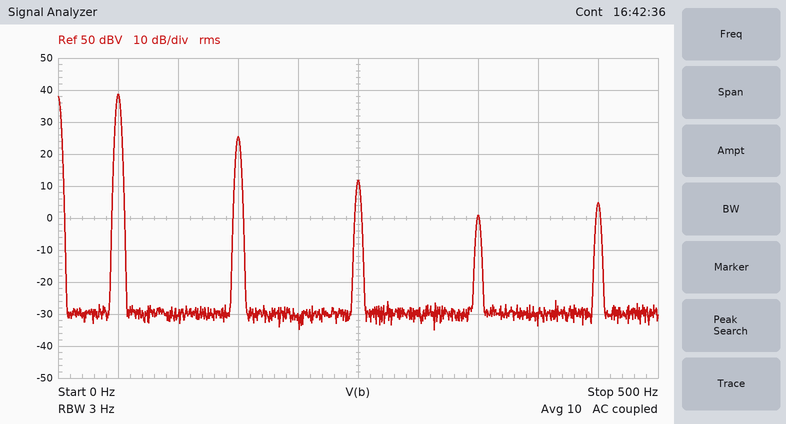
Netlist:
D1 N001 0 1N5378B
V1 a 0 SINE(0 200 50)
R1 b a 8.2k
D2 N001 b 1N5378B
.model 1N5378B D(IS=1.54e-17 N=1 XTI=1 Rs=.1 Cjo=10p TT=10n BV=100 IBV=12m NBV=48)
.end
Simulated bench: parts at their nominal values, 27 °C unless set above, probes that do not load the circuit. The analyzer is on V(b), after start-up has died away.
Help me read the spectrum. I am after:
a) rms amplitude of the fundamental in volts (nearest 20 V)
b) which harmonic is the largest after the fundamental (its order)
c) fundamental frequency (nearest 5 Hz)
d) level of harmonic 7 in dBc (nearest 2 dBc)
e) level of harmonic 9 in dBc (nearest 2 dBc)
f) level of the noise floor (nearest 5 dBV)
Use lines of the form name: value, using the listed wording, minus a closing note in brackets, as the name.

rms amplitude of the fundamental in volts: 80 V
which harmonic is the largest after the fundamental: 3
fundamental frequency: 50 Hz
level of harmonic 7 in dBc: -38 dBc
level of harmonic 9 in dBc: -34 dBc
level of the noise floor: -30 dBV
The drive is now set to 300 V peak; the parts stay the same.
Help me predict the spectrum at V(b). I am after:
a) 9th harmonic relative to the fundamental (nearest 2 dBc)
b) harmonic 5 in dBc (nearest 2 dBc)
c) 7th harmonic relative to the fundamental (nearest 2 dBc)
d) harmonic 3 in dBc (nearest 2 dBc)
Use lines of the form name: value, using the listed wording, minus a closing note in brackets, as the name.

9th harmonic relative to the fundamental: -46 dBc
harmonic 5 in dBc: -18 dBc
7th harmonic relative to the fundamental: -28 dBc
harmonic 3 in dBc: -12 dBc
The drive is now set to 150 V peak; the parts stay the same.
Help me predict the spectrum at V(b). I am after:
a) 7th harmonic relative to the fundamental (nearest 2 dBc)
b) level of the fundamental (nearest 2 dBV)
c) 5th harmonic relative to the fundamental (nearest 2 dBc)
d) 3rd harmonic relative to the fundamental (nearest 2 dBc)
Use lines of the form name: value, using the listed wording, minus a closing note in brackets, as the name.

7th harmonic relative to the fundamental: -32 dBc
level of the fundamental: 38 dBV
5th harmonic relative to the fundamental: -38 dBc
3rd harmonic relative to the fundamental: -16 dBc
